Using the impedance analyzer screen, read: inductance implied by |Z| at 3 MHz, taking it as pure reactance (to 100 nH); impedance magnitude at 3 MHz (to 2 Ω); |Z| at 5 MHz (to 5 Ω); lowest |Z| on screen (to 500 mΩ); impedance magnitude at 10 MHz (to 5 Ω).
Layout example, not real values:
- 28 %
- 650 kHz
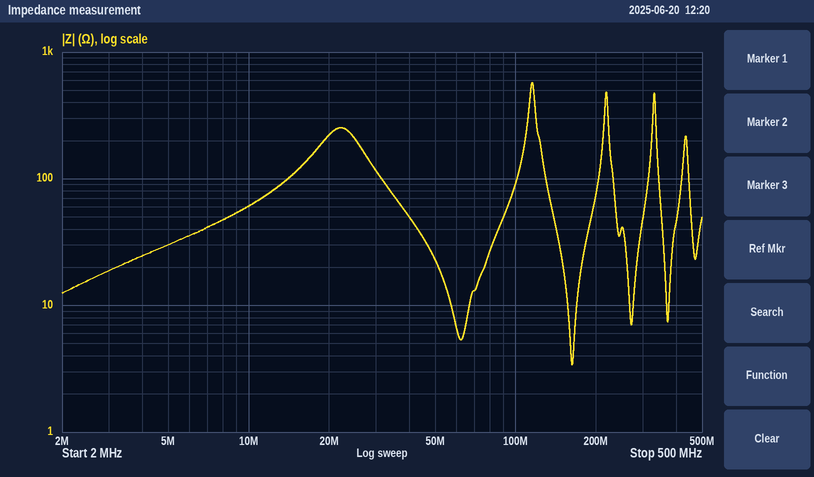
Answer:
- 1.0 µH
- 18 Ω
- 30 Ω
- 3.5 Ω
- 60 Ω
